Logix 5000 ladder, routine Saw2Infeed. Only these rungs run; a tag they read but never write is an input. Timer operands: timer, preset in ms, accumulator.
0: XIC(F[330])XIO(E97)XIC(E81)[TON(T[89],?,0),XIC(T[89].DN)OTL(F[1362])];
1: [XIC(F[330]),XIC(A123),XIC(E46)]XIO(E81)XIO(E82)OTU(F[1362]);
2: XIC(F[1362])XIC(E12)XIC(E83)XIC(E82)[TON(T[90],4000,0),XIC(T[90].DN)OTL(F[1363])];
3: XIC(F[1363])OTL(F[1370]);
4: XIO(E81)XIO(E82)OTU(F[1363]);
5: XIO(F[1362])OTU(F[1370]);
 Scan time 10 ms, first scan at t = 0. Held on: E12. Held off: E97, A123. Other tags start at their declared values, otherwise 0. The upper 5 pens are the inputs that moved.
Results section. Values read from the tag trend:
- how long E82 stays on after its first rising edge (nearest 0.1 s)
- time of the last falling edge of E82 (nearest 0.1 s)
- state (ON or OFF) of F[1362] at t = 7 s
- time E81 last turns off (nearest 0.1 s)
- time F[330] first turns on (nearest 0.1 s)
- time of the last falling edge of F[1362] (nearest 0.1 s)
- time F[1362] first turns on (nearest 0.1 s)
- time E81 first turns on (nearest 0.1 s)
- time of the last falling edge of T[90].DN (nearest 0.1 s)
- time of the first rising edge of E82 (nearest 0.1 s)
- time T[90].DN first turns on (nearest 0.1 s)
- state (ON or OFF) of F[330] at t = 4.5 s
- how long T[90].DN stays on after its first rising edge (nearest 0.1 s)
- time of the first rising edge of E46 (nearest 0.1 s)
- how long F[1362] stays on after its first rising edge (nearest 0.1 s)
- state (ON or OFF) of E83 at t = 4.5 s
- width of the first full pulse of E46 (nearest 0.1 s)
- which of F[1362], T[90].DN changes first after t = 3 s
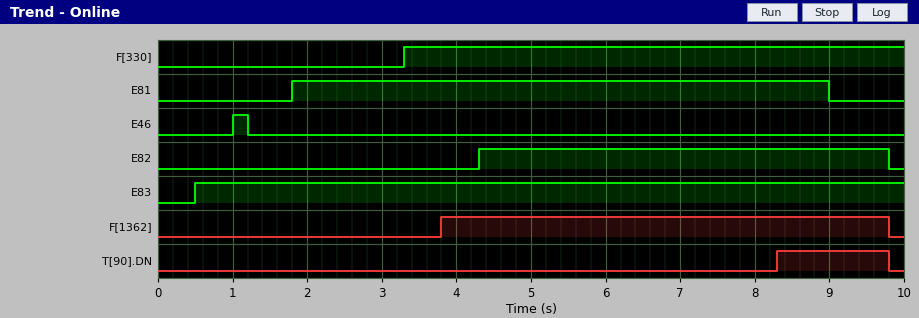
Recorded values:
5.5 s
9.8 s
ON
9.0 s
3.3 s
9.8 s
3.8 s
1.8 s
9.8 s
4.3 s
8.3 s
ON
1.5 s
1.0 s
6.0 s
ON
0.2 s
F[1362]
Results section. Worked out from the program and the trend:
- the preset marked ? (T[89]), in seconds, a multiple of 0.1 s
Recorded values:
0.5 s
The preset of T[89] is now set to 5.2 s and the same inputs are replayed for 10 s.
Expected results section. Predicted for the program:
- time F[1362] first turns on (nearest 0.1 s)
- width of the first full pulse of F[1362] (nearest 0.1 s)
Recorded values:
8.5 s
1.3 s
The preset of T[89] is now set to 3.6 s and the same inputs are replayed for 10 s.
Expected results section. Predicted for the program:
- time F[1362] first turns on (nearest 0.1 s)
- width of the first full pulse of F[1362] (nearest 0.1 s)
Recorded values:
6.9 s
2.9 s
